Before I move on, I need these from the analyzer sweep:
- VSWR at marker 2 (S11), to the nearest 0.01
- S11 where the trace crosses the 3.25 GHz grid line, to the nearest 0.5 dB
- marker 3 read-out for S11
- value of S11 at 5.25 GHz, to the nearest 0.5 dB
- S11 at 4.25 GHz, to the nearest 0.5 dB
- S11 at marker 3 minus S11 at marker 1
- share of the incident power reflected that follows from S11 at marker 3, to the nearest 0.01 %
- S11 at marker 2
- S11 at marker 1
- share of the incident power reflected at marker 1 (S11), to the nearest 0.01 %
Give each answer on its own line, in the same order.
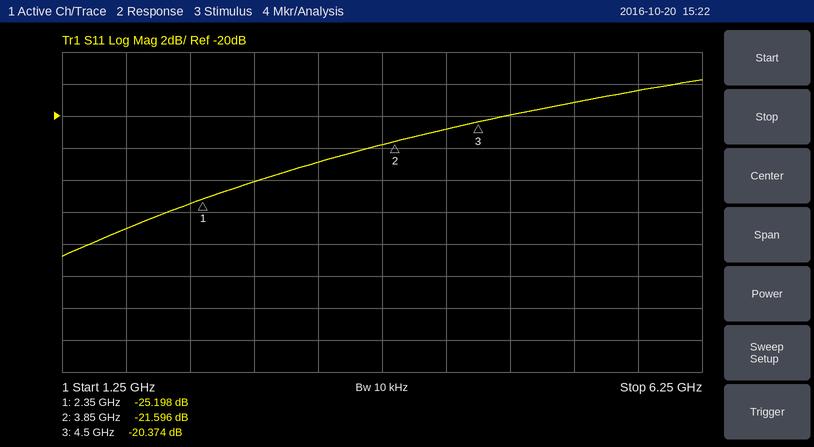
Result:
1.18
-23.0 dB
-20.374 dB
-19.0 dB
-21.0 dB
4.824 dB
0.92 %
-21.596 dB
-25.198 dB
0.30 %
